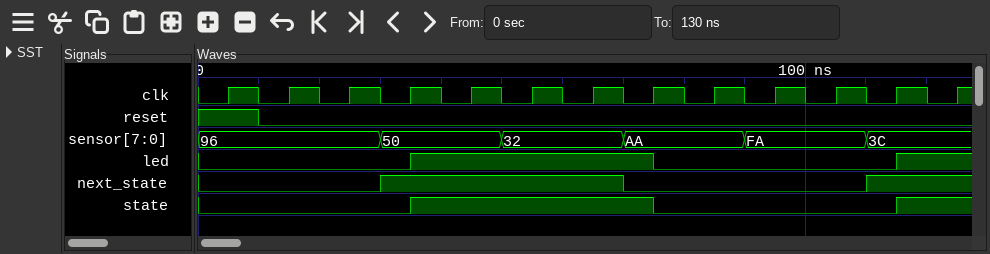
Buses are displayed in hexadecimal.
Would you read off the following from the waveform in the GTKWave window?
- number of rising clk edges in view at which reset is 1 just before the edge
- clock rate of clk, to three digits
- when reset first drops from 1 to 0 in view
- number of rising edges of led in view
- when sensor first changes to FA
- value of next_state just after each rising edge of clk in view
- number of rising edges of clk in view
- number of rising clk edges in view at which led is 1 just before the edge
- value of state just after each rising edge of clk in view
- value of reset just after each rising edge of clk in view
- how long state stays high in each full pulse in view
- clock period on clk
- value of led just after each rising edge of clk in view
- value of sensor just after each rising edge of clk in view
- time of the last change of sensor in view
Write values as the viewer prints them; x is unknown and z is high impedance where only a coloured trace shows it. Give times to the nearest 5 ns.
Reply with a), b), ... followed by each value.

a) 1
b) 100 MHz
c) 10 ns
d) 2
e) 90 ns
f) 0 0 0 1 1 1 1 0 0 0 0 1 1
g) 13
h) 5
i) 0 0 0 1 1 1 1 0 0 0 0 1 1
j) 1 0 0 0 0 0 0 0 0 0 0 0 0
k) 40 ns
l) 10 ns
m) 0 0 0 1 1 1 1 0 0 0 0 1 1
n) 96, 96, 96, 50, 50, 32, 32, AA, AA, FA, FA, 3C, 3C
o) 110 ns
